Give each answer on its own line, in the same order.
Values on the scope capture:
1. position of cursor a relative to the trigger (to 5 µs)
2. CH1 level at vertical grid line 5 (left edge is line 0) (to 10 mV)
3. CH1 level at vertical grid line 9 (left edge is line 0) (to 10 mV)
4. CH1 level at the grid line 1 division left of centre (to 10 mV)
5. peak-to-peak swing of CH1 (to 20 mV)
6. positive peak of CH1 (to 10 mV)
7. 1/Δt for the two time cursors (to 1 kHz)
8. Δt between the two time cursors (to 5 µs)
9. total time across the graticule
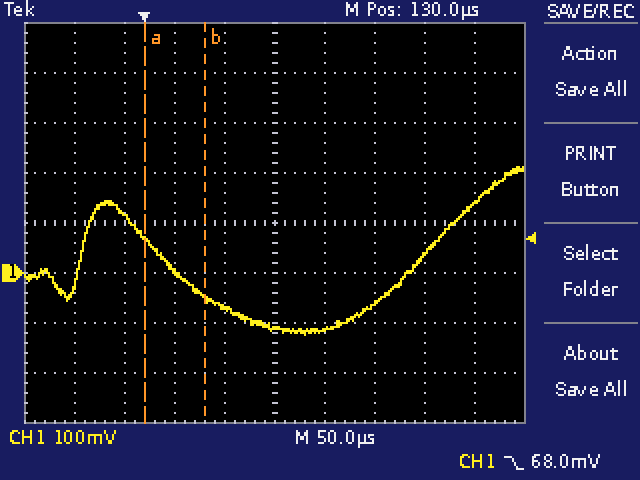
0 µs
-110 mV
140 mV
-70 mV
340 mV
210 mV
17 kHz
60 µs
500 µs
